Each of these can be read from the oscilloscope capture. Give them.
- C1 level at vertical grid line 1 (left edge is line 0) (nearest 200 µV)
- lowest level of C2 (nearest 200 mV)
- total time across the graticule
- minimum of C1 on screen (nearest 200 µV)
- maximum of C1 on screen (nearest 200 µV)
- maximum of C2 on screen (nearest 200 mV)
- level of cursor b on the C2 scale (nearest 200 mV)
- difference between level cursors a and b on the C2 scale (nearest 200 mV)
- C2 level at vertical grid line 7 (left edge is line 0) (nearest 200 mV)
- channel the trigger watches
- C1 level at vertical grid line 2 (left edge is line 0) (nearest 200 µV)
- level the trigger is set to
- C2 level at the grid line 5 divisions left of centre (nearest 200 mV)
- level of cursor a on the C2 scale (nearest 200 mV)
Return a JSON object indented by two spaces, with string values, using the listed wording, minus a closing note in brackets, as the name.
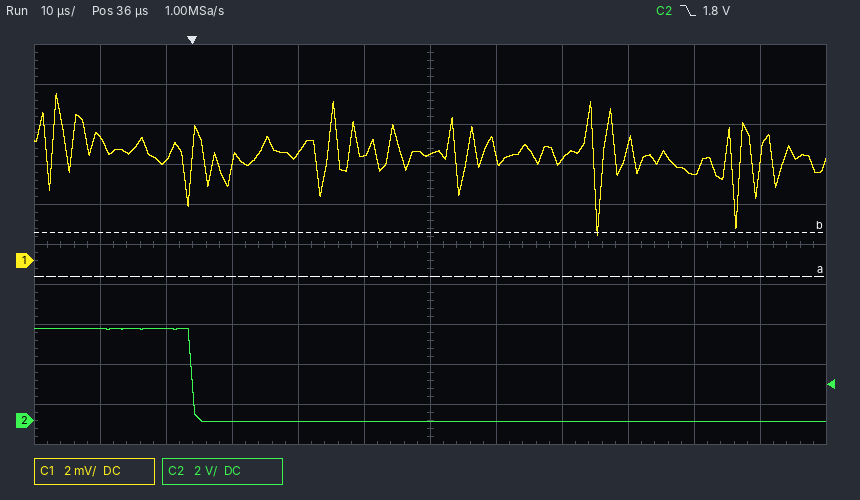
{
  "C1 level at vertical grid line 1 (left edge is line 0)": "6.2 mV",
  "lowest level of C2": "0.0 V",
  "total time across the graticule": "120 µs",
  "minimum of C1 on screen": "1.2 mV",
  "maximum of C1 on screen": "8.4 mV",
  "maximum of C2 on screen": "4.6 V",
  "level of cursor b on the C2 scale": "9.4 V",
  "difference between level cursors a and b on the C2 scale": "2.2 V",
  "C2 level at vertical grid line 7 (left edge is line 0)": "0.0 V",
  "channel the trigger watches": "C2",
  "C1 level at vertical grid line 2 (left edge is line 0)": "5.0 mV",
  "level the trigger is set to": "1.8 V",
  "C2 level at the grid line 5 divisions left of centre": "4.6 V",
  "level of cursor a on the C2 scale": "7.2 V"
}
